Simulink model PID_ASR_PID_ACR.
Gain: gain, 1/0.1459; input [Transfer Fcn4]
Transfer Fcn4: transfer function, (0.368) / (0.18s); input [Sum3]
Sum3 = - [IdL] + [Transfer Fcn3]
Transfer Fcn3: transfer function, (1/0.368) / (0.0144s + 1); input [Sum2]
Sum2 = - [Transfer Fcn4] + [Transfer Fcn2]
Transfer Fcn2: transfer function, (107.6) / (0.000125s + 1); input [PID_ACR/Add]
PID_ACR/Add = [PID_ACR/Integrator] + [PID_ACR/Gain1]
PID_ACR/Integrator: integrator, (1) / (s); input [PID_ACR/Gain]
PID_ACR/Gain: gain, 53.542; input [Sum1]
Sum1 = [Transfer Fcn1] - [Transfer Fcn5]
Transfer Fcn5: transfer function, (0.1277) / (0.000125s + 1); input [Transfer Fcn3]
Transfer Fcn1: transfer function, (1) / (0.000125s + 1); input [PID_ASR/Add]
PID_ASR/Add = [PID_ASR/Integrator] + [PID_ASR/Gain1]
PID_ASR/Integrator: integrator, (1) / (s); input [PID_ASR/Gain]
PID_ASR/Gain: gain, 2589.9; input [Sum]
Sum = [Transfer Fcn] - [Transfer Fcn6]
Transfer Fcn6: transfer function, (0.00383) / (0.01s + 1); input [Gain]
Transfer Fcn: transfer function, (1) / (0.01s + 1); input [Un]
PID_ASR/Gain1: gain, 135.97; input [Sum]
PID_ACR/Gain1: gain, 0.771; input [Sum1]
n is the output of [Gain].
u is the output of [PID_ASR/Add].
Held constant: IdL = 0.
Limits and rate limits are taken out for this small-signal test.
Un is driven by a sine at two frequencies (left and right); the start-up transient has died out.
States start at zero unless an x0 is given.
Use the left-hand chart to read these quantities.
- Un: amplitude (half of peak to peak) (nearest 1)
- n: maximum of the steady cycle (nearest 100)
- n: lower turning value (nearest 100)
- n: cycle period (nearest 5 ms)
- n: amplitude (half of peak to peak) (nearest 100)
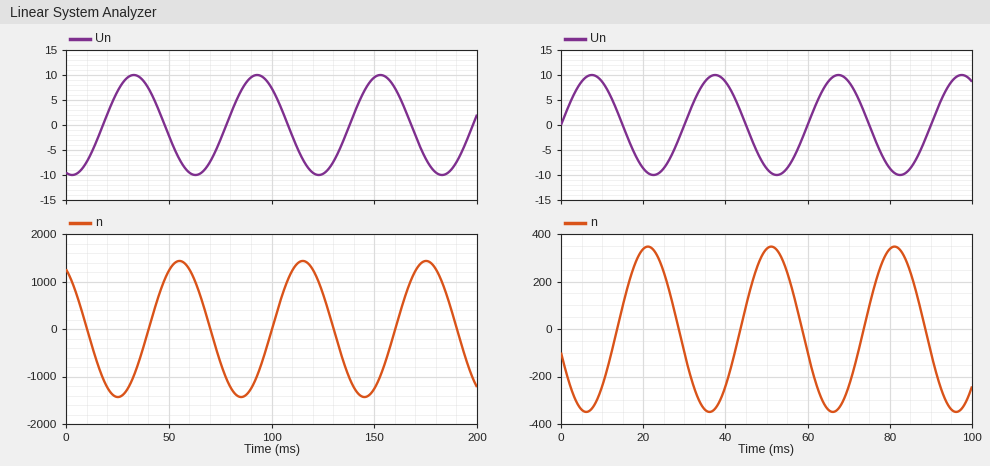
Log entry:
10
1400
-1400
60 ms
1400
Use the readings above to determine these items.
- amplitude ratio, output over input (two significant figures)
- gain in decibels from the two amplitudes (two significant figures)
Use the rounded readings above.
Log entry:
140
43 dB
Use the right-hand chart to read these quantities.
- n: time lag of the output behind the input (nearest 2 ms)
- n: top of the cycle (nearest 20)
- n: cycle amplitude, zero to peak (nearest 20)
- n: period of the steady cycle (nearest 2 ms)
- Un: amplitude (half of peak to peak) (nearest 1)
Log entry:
14 ms
340
340
30 ms
10
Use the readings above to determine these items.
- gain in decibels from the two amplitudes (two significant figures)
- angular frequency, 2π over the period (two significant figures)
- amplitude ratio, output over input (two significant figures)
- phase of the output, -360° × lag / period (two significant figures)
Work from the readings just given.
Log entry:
31 dB
0.21 rad/ms
34
-170°
